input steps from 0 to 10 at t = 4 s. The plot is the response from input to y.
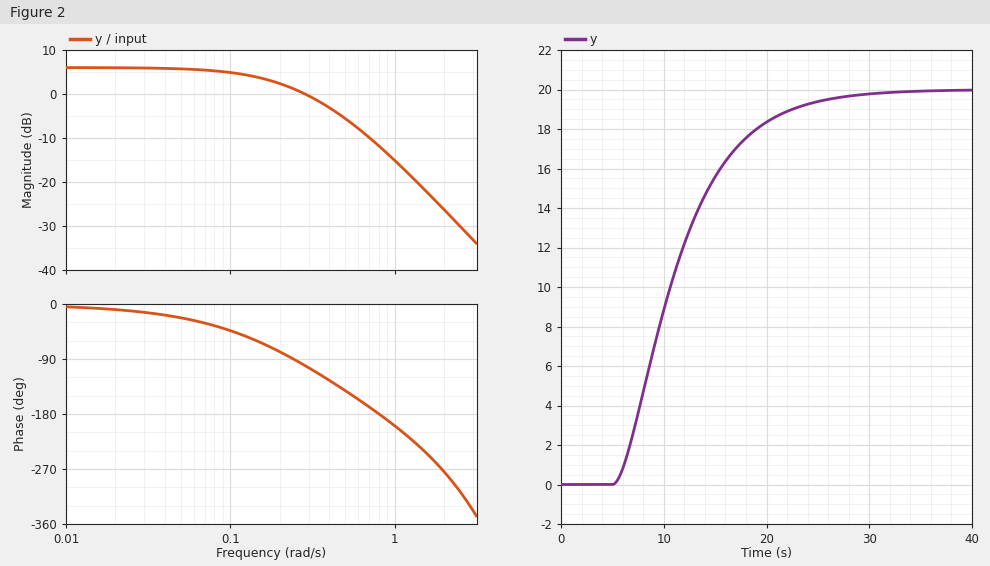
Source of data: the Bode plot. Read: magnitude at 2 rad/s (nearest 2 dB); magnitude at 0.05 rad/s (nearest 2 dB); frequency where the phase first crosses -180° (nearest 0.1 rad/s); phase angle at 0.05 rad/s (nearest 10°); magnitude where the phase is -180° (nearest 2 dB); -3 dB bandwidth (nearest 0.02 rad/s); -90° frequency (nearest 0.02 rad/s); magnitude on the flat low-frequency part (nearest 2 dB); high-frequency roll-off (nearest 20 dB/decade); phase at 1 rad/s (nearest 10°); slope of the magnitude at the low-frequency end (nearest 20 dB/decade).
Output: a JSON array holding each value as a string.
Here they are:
["-26 dB", "6 dB", "0.8 rad/s", "-20°", "-12 dB", "0.18 rad/s", "0.24 rad/s", "6 dB", "-40 dB/decade", "-200°", "0 dB/decade"]
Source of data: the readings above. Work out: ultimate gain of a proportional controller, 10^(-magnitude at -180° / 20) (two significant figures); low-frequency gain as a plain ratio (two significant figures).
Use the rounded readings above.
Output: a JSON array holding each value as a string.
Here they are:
["4.0", "2.0"]
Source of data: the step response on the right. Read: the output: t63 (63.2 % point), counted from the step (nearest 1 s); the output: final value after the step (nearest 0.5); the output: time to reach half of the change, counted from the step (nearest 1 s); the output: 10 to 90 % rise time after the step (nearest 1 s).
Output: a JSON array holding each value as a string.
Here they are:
["8 s", "20.0", "7 s", "12 s"]
